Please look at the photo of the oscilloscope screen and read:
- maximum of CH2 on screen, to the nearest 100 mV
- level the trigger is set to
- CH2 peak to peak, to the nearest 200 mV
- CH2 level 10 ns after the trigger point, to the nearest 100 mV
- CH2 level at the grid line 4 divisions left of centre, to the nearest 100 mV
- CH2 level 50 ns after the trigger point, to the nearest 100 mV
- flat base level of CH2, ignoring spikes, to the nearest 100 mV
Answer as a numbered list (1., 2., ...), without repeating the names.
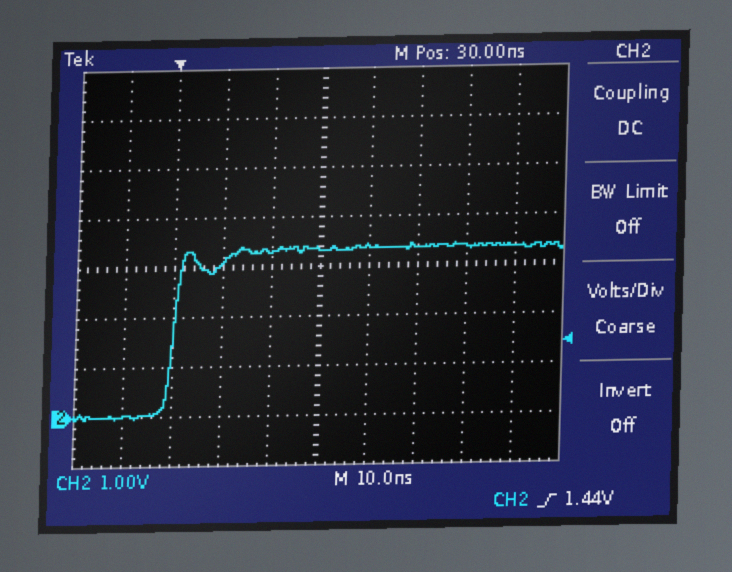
1. 3.4 V
2. 1.44 V
3. 3.4 V
4. 3.1 V
5. 0.0 V
6. 3.4 V
7. 0.0 V
